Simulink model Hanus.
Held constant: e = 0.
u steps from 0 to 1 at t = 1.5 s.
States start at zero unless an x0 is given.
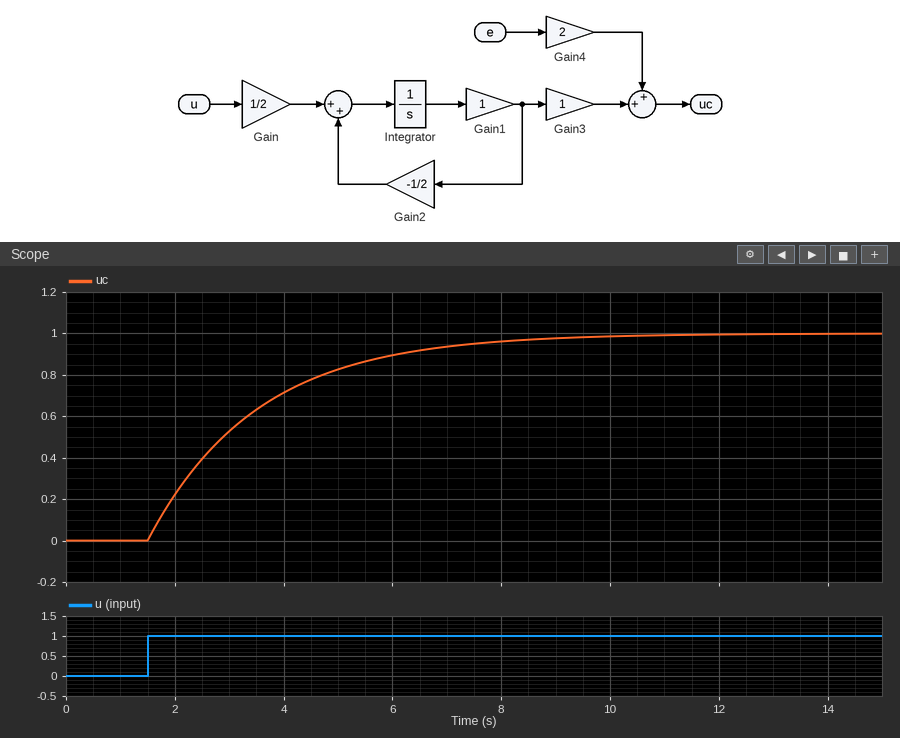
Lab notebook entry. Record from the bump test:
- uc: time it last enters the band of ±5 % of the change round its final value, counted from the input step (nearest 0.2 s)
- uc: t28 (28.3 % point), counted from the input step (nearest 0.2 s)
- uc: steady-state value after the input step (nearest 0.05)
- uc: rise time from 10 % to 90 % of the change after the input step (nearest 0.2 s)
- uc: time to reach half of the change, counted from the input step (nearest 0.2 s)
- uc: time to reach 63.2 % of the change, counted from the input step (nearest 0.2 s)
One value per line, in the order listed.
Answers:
6.0 s
0.6 s
1.00
4.4 s
1.4 s
2.0 s
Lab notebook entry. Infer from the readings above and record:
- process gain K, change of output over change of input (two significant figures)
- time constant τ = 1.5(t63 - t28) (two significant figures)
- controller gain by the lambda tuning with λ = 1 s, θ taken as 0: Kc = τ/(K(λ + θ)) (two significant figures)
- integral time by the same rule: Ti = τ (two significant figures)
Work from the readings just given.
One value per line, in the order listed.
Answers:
1.0
2.1 s
2.1
2.1 s
